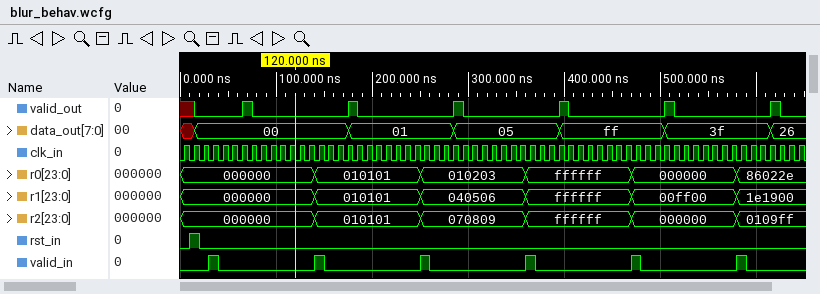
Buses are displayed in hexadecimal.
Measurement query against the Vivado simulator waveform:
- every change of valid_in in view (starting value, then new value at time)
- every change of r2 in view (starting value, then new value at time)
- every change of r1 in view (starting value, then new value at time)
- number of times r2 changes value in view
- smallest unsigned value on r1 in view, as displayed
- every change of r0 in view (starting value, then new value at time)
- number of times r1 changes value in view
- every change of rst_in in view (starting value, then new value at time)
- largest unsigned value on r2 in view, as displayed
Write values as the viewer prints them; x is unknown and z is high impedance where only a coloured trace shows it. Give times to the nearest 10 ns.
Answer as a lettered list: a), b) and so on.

a) 0, 1 at 30 ns, 0 at 40 ns, 1 at 140 ns, 0 at 150 ns, 1 at 250 ns, 0 at 260 ns, 1 at 360 ns, 0 at 370 ns, 1 at 470 ns, 0 at 480 ns, 1 at 580 ns, 0 at 590 ns
b) 000000, 010101 at 140 ns, 070809 at 250 ns, ffffff at 360 ns, 000000 at 470 ns, 0109ff at 580 ns
c) 000000, 010101 at 140 ns, 040506 at 250 ns, ffffff at 360 ns, 00ff00 at 470 ns, 1e1900 at 580 ns
d) 5
e) 000000
f) 000000, 010101 at 140 ns, 010203 at 250 ns, ffffff at 360 ns, 000000 at 470 ns, 86022e at 580 ns
g) 5
h) 0, 1 at 10 ns, 0 at 20 ns
i) ffffff
